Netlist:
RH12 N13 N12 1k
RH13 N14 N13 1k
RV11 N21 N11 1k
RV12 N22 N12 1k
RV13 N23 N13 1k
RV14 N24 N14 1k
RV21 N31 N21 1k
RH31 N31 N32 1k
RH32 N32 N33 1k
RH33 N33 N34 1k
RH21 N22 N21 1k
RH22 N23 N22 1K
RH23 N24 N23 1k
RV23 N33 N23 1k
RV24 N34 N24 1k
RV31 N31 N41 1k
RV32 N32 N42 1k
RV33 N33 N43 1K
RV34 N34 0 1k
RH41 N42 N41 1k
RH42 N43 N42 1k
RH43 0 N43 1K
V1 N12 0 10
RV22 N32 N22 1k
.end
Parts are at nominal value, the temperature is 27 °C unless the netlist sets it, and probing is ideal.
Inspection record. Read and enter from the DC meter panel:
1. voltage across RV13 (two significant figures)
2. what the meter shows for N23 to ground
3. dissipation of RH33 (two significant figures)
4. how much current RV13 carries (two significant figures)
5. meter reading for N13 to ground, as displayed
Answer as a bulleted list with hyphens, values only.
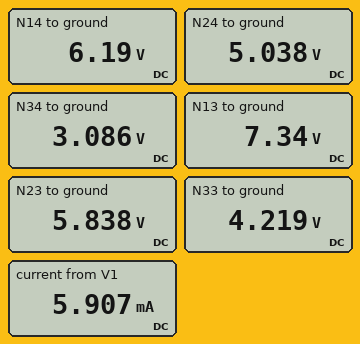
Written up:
- 1.5 V
- 5.838 V
- 1.3 mW
- 1.5 mA
- 7.34 V
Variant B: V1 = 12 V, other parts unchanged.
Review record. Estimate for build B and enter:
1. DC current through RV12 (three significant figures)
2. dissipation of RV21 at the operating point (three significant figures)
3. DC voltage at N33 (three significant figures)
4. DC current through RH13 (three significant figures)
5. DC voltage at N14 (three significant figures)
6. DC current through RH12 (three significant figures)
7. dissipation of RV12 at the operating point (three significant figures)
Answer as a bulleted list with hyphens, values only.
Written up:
- 3.90 mA
- 742 µW
- 5.06 V
- 1.38 mA
- 7.43 V
- 3.19 mA
- 15.2 mW
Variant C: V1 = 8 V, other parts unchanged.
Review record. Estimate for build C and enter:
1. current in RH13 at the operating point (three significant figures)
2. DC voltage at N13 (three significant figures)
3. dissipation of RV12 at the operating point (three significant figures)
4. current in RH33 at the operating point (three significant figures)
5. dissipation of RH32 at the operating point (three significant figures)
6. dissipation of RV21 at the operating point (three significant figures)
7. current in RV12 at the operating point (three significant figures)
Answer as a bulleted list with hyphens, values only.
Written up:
- 922 µA
- 5.87 V
- 6.76 mW
- 907 µA
- 534 µW
- 330 µW
- 2.60 mA
